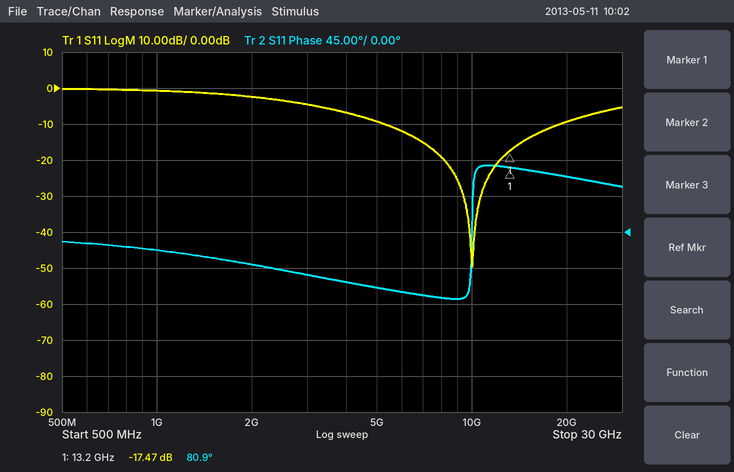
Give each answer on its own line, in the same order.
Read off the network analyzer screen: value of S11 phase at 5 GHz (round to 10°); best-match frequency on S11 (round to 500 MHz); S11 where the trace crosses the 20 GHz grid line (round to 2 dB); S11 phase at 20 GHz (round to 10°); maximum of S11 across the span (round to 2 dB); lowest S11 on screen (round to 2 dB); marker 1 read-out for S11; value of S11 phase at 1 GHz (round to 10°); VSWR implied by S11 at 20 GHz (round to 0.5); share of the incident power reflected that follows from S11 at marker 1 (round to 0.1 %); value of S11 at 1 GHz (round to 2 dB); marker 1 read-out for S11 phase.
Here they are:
-70°
10.0 GHz
-10 dB
70°
0 dB
-50 dB
-17.47 dB
-20°
2.0
1.8 %
0 dB
80.9°
